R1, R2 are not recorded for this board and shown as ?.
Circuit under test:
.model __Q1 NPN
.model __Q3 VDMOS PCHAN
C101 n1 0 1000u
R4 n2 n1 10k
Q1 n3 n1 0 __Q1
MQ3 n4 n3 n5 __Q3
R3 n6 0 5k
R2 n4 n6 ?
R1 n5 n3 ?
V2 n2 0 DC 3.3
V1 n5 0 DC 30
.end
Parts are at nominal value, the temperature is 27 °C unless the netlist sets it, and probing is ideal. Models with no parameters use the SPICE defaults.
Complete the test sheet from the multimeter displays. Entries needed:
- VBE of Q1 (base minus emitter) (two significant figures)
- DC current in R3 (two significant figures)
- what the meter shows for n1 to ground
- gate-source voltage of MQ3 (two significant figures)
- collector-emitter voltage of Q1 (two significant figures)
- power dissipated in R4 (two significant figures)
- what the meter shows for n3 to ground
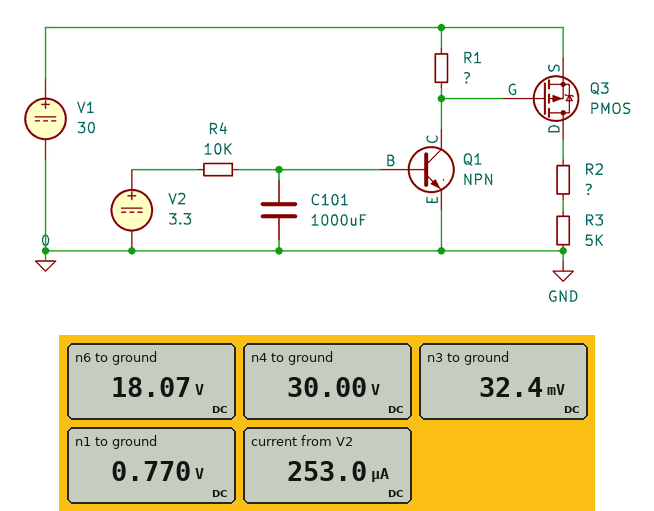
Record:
770 mV
3.6 mA
0.770 V
-30 V
32 mV
640 µW
32.4 mV
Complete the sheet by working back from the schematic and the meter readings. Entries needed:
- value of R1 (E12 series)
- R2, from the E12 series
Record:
82 kΩ
3.3 kΩ
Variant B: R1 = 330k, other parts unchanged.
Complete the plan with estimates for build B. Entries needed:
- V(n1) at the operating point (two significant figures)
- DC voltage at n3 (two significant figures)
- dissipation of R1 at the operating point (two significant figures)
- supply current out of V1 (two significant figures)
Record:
760 mV
22 mV
2.7 mW
3.7 mA
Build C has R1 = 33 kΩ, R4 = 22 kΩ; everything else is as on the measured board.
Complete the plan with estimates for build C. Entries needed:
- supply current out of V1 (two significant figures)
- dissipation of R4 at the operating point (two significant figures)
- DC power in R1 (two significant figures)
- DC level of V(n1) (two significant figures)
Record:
4.5 mA
290 µW
27 mW
780 mV
